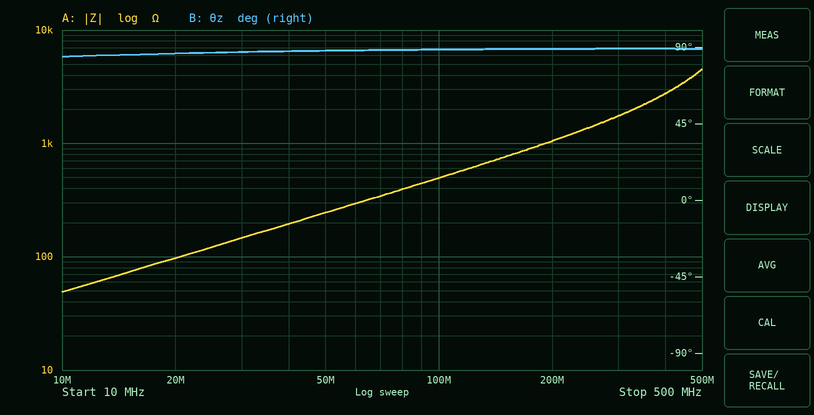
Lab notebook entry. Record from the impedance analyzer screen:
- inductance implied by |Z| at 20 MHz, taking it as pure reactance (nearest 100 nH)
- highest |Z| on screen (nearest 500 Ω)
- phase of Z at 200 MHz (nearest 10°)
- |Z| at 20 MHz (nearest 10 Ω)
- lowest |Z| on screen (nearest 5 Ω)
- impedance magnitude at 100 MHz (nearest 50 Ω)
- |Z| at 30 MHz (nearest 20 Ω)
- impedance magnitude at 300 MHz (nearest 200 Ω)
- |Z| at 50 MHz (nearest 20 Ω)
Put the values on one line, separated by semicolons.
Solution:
800 nH; 4.5 kΩ; 90°; 100 Ω; 50 Ω; 500 Ω; 140 Ω; 1.8 kΩ; 240 Ω
